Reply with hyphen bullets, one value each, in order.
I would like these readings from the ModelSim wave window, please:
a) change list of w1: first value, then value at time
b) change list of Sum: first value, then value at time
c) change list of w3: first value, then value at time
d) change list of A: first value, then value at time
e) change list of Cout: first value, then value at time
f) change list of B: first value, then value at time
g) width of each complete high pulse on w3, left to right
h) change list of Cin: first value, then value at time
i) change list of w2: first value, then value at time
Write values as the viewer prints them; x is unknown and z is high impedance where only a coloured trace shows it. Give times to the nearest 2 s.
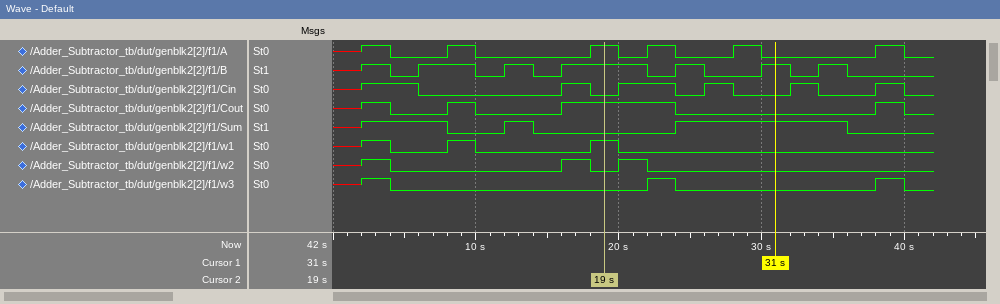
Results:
- x, 1 at 2 s, 0 at 4 s, 1 at 8 s, 0 at 10 s, 1 at 18 s, 0 at 20 s
- x, 1 at 2 s, 0 at 8 s, 1 at 12 s, 0 at 14 s, 1 at 24 s, 0 at 36 s
- x, 1 at 2 s, 0 at 4 s, 1 at 22 s, 0 at 24 s, 1 at 38 s, 0 at 40 s
- x, 1 at 2 s, 0 at 4 s, 1 at 8 s, 0 at 10 s, 1 at 18 s, 0 at 20 s, 1 at 22 s, 0 at 24 s, 1 at 28 s, 0 at 30 s, 1 at 38 s, 0 at 40 s
- x, 1 at 2 s, 0 at 4 s, 1 at 8 s, 0 at 10 s, 1 at 16 s, 0 at 24 s, 1 at 38 s, 0 at 40 s
- x, 1 at 2 s, 0 at 4 s, 1 at 6 s, 0 at 10 s, 1 at 12 s, 0 at 14 s, 1 at 16 s, 0 at 22 s, 1 at 24 s, 0 at 26 s, 1 at 30 s, 0 at 32 s, 1 at 34 s, 0 at 36 s
- 2 s, 2 s
- x, 1 at 2 s, 0 at 6 s, 1 at 16 s, 0 at 18 s, 1 at 20 s, 0 at 24 s, 1 at 26 s, 0 at 28 s, 1 at 32 s, 0 at 34 s, 1 at 38 s, 0 at 40 s
- x, 1 at 2 s, 0 at 4 s, 1 at 16 s, 0 at 18 s, 1 at 20 s, 0 at 22 s
